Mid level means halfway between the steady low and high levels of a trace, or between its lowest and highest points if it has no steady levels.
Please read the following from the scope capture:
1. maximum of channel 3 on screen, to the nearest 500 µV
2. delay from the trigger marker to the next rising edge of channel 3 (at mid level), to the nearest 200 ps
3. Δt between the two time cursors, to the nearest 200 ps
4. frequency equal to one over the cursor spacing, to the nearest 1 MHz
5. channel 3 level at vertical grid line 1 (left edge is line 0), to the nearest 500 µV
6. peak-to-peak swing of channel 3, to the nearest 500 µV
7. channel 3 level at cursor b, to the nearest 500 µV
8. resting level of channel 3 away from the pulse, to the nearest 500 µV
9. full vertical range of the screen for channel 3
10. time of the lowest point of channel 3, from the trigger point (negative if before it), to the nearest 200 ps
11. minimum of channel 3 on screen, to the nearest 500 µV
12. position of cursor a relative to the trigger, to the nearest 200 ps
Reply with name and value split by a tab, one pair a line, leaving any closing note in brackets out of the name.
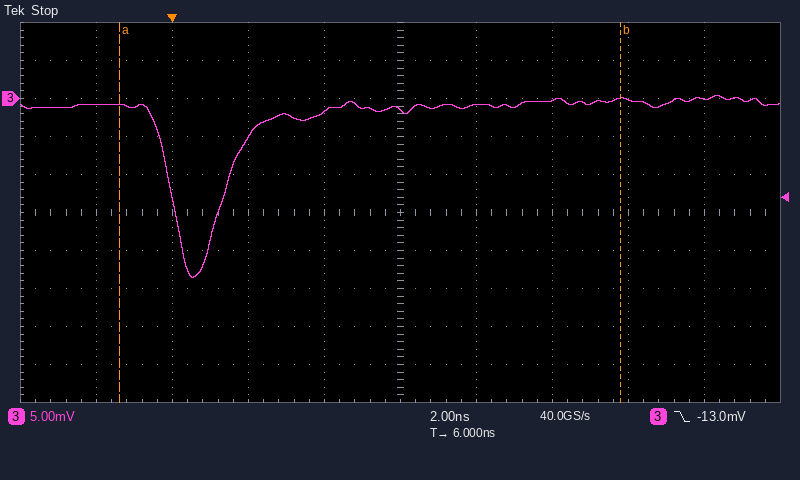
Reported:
maximum of channel 3 on screen, to the nearest 500 µV	500 µV
delay from the trigger marker to the next rising edge of channel 3 (at mid level), to the nearest 200 ps	1.4 ns
Δt between the two time cursors, to the nearest 200 ps	13.2 ns
frequency equal to one over the cursor spacing, to the nearest 1 MHz	76 MHz
channel 3 level at vertical grid line 1 (left edge is line 0), to the nearest 500 µV	-1.0 mV
peak-to-peak swing of channel 3, to the nearest 500 µV	24.0 mV
channel 3 level at cursor b, to the nearest 500 µV	0.0 mV
resting level of channel 3 away from the pulse, to the nearest 500 µV	-1.0 mV
full vertical range of the screen for channel 3	50 mV
time of the lowest point of channel 3, from the trigger point (negative if before it), to the nearest 200 ps	+600 ps
minimum of channel 3 on screen, to the nearest 500 µV	-23.5 mV
position of cursor a relative to the trigger, to the nearest 200 ps	-1.4 ns
